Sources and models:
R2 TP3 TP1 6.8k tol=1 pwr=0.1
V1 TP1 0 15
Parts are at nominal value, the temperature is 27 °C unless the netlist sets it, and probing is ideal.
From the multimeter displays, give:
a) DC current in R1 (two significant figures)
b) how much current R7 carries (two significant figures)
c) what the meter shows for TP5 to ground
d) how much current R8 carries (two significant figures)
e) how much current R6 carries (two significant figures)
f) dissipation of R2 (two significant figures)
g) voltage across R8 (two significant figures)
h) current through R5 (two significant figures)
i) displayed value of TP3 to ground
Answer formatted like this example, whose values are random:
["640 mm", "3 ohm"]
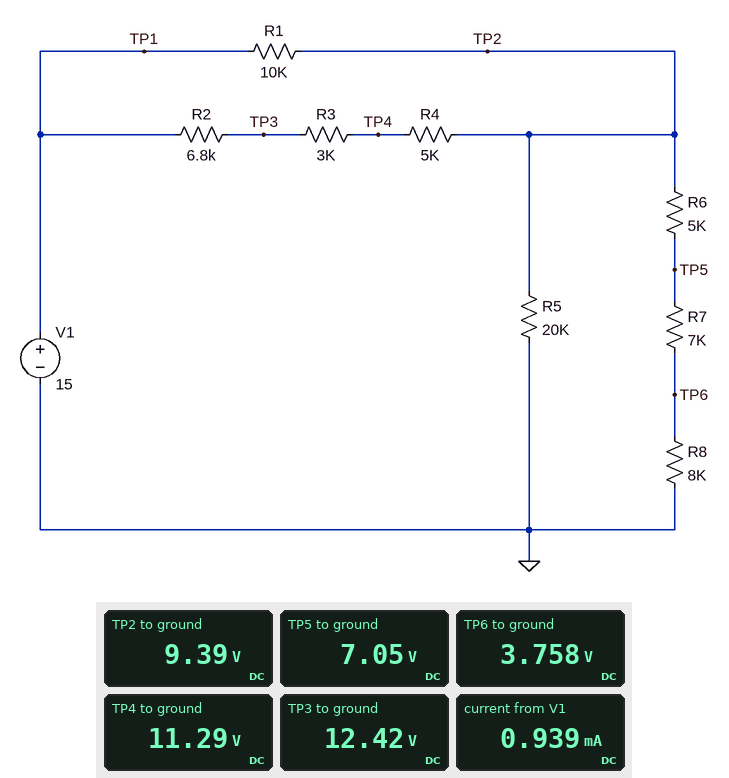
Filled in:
["560 µA", "470 µA", "7.05 V", "470 µA", "470 µA", "980 µW", "3.8 V", "470 µA", "12.42 V"]
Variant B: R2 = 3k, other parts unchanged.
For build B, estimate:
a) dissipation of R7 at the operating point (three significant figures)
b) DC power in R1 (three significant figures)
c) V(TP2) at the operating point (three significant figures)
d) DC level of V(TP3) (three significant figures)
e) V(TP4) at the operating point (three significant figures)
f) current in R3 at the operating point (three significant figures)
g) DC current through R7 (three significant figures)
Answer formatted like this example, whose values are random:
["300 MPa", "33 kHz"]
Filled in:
["1.70 mW", "2.66 mW", "9.84 V", "13.6 V", "12.2 V", "469 µA", "492 µA"]
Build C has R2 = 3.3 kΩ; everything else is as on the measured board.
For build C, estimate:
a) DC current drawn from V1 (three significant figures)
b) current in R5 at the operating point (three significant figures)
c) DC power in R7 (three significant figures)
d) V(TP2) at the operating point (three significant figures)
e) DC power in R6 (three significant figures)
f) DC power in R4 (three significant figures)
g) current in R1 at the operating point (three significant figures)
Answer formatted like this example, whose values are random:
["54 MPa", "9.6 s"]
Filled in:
["980 µA", "490 µA", "1.68 mW", "9.80 V", "1.20 mW", "1.06 mW", "520 µA"]
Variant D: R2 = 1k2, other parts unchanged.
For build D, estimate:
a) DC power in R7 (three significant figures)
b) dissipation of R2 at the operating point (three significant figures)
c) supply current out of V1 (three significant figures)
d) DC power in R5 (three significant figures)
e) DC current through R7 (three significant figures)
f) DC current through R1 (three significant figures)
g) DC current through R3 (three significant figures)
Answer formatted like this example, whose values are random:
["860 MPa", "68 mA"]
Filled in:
["1.80 mW", "335 µW", "1.01 mA", "5.14 mW", "507 µA", "486 µA", "528 µA"]
